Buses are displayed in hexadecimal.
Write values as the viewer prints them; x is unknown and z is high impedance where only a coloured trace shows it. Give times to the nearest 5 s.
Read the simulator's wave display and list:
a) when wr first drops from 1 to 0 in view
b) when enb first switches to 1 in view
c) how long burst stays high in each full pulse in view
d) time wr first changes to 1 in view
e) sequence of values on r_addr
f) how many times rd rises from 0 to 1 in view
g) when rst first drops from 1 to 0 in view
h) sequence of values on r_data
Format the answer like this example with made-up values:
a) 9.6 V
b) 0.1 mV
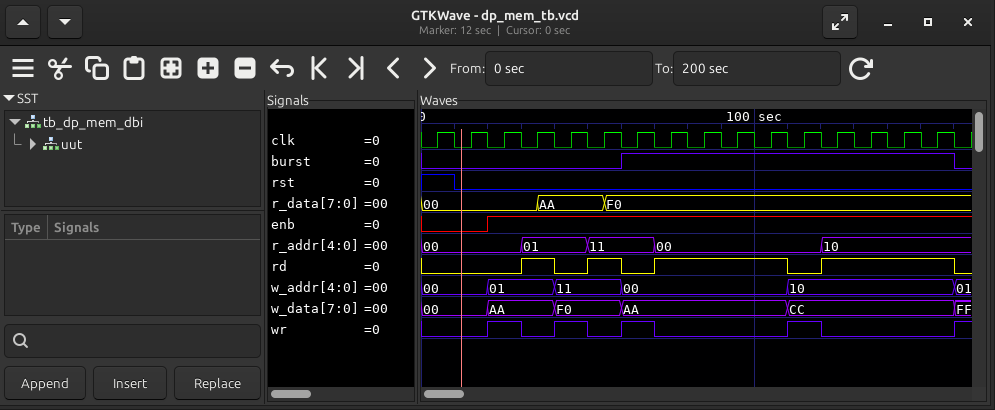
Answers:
a) 30 s
b) 20 s
c) 100 s
d) 20 s
e) 00, 01, 11, 00, 10
f) 4
g) 10 s
h) 00, AA, F0
